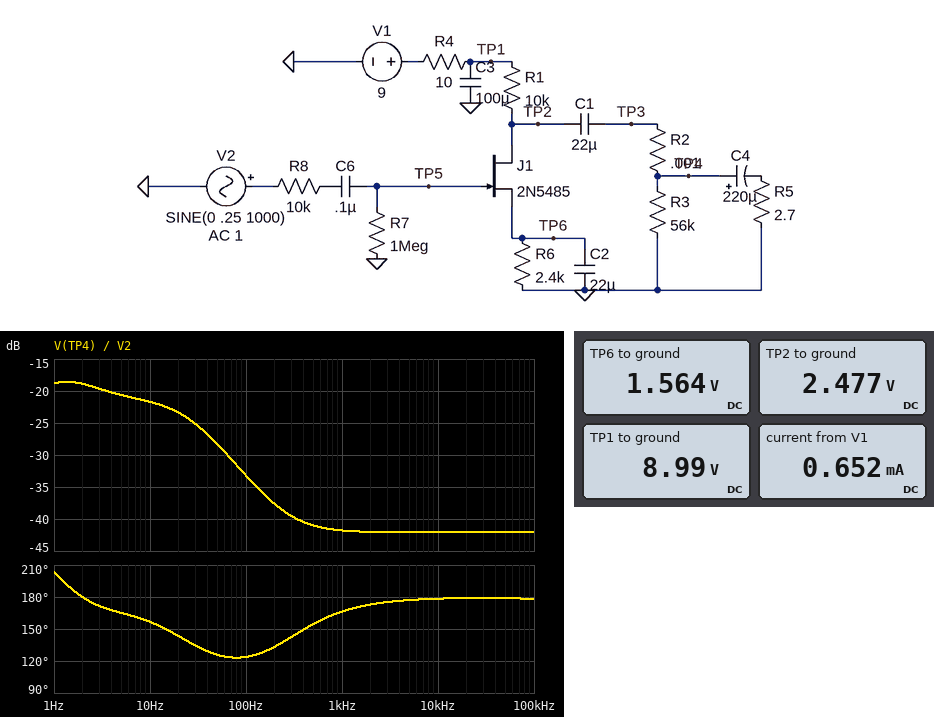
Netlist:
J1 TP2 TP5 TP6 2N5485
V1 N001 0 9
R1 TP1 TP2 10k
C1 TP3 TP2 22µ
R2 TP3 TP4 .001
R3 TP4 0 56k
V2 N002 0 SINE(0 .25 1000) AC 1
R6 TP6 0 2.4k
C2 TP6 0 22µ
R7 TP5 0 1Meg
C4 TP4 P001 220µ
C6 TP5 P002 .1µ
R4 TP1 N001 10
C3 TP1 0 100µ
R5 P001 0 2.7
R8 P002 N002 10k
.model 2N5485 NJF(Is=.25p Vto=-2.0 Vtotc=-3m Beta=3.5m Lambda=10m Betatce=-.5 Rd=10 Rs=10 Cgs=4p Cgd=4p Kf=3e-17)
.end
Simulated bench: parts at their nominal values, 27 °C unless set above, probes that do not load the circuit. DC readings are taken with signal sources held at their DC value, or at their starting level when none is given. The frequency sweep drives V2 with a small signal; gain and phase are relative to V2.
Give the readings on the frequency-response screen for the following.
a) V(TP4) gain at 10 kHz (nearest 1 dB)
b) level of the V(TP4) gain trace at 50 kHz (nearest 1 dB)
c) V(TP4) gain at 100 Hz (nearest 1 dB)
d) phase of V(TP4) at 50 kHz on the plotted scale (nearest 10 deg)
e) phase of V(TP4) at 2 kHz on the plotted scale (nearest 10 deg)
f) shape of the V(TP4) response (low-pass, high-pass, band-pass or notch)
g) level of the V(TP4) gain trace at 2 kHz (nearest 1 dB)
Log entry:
-42 dB
-42 dB
-33 dB
180 deg
170 deg
low-pass
-42 dB
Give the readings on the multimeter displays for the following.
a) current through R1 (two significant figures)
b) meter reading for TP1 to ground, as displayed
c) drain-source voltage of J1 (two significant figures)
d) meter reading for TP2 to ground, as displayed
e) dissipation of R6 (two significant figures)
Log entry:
650 µA
8.99 V
910 mV
2.477 V
1.0 mW
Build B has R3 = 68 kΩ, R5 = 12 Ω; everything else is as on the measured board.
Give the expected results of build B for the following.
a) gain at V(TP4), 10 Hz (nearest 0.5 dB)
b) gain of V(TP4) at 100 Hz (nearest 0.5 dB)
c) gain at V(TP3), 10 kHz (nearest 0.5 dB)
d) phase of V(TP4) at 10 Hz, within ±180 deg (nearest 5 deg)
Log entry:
-21.5 dB
-28.0 dB
-29.0 dB
165 deg
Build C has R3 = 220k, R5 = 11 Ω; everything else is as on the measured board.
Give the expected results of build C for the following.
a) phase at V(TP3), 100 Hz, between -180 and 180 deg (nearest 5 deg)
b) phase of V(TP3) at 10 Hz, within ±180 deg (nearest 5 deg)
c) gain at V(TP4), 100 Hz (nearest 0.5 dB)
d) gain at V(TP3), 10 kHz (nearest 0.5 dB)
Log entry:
160 deg
165 deg
-28.5 dB
-30.0 dB
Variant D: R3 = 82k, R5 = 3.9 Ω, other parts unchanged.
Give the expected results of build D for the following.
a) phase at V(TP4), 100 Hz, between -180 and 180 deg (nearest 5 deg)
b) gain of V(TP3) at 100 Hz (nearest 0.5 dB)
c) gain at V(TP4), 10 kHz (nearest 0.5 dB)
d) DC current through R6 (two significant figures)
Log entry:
130 deg
-32.5 dB
-39.0 dB
650 µA
